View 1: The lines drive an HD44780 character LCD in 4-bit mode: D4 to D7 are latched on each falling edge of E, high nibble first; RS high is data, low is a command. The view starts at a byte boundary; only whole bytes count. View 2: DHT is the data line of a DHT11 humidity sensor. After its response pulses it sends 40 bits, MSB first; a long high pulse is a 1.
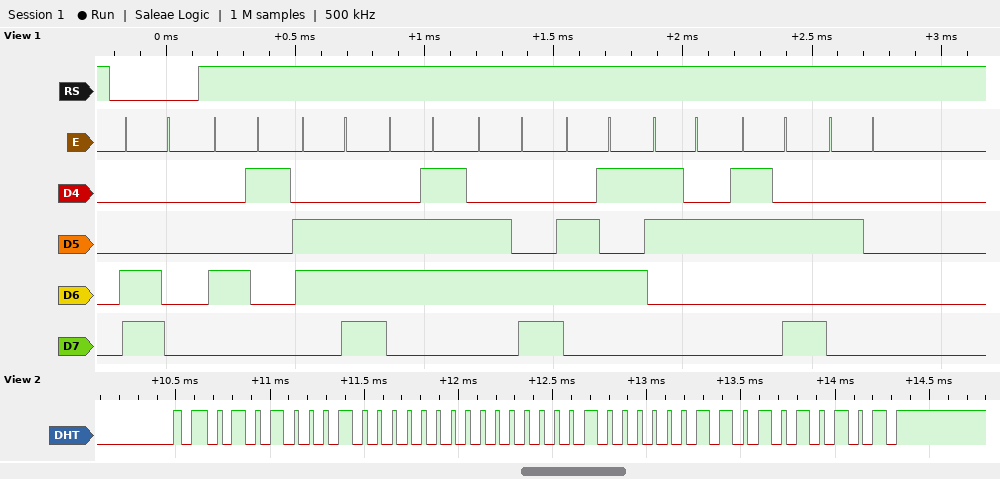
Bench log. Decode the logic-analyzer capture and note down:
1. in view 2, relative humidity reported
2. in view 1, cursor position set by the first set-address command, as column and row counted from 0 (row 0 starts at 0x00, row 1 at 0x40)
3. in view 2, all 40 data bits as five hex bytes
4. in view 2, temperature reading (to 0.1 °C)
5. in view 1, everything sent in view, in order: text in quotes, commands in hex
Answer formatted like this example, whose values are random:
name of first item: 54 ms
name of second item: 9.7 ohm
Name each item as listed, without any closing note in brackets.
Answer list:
in view 2, relative humidity reported: 81 %
in view 1, cursor position set by the first set-address command, as column and row counted from 0: column 0, row 1
in view 2, all 40 data bits as five hex bytes: 51 00 01 03 55
in view 2, temperature reading: 1.3 °C
in view 1, everything sent in view, in order: text in quotes, commands in hex: 0xC0 "Angle2: "
